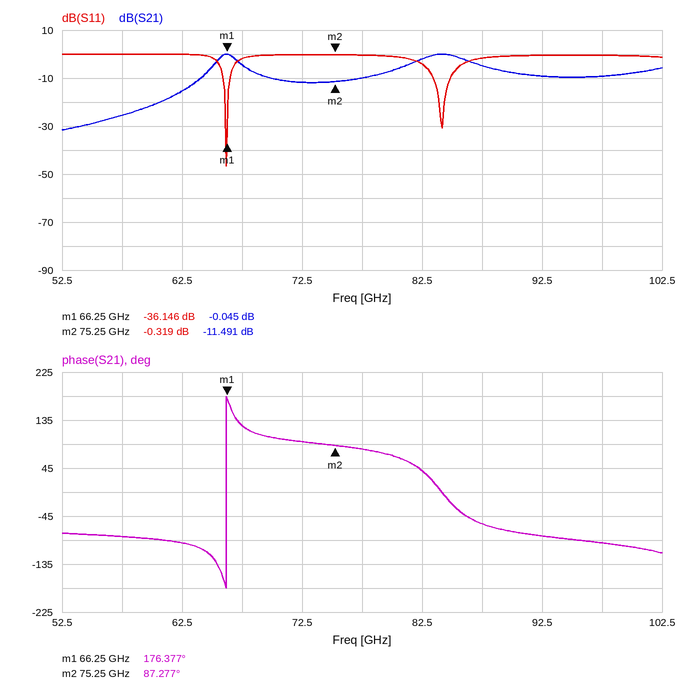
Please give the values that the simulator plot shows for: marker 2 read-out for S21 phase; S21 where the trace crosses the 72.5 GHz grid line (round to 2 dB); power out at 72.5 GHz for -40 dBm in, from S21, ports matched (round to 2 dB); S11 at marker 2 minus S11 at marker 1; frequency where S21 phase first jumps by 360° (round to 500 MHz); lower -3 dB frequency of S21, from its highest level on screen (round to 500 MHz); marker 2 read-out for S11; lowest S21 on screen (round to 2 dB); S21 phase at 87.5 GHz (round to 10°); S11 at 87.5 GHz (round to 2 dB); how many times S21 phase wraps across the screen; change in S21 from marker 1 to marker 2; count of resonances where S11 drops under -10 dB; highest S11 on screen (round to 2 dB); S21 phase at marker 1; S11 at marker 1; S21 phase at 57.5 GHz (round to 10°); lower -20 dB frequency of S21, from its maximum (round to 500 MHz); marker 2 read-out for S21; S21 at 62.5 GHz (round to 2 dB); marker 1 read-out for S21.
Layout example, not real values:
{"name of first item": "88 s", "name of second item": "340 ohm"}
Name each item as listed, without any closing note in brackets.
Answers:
{"marker 2 read-out for S21 phase": "87.277°", "S21 where the trace crosses the 72.5 GHz grid line": "-12 dB", "power out at 72.5 GHz for -40 dBm in, from S21, ports matched": "-52 dBm", "S11 at marker 2 minus S11 at marker 1": "35.827 dB", "frequency where S21 phase first jumps by 360°": "66.0 GHz", "lower -3 dB frequency of S21, from its highest level on screen": "65.5 GHz", "marker 2 read-out for S11": "-0.319 dB", "lowest S21 on screen": "-32 dB", "S21 phase at 87.5 GHz": "-60°", "S11 at 87.5 GHz": "-2 dB", "how many times S21 phase wraps across the screen": "1", "change in S21 from marker 1 to marker 2": "-11.446 dB", "count of resonances where S11 drops under -10 dB": "2", "highest S11 on screen": "0 dB", "S21 phase at marker 1": "176.377°", "S11 at marker 1": "-36.146 dB", "S21 phase at 57.5 GHz": "-80°", "lower -20 dB frequency of S21, from its maximum": "60.5 GHz", "marker 2 read-out for S21": "-11.491 dB", "S21 at 62.5 GHz": "-16 dB", "marker 1 read-out for S21": "-0.045 dB"}
